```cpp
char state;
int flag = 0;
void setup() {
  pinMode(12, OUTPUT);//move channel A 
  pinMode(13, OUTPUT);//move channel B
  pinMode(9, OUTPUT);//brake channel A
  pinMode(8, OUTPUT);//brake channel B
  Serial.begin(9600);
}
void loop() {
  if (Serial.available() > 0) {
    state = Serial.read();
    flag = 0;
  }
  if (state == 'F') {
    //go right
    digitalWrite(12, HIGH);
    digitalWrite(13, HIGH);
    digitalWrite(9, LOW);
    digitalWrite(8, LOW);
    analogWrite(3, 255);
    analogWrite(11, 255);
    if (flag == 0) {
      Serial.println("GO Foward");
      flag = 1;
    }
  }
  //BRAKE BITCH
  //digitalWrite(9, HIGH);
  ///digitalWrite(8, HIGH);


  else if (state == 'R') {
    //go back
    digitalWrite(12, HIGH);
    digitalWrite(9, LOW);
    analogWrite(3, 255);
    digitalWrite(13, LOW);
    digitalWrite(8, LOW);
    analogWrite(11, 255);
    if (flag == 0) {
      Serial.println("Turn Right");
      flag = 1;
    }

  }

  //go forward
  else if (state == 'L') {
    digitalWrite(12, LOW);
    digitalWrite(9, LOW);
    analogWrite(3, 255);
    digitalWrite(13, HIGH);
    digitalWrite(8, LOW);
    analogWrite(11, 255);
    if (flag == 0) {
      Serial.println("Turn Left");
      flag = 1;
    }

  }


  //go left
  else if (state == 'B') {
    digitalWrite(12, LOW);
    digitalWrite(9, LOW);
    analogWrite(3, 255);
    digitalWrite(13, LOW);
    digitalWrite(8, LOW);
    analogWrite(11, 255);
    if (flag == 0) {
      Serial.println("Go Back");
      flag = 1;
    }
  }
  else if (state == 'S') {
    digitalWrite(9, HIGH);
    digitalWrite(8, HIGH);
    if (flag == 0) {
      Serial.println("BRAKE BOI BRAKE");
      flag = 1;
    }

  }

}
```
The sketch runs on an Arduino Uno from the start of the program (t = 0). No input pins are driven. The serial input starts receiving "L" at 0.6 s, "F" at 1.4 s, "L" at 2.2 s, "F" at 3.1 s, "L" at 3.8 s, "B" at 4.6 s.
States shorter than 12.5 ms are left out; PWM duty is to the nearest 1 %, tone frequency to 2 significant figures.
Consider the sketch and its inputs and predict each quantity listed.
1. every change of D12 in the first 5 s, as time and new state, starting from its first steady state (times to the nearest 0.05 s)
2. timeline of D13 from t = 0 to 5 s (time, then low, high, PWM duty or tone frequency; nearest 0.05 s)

0 s low; 1.4 s high; 2.2 s low; 3.1 s high; 3.8 s low
0 s low; 0.6 s high; 4.6 s low
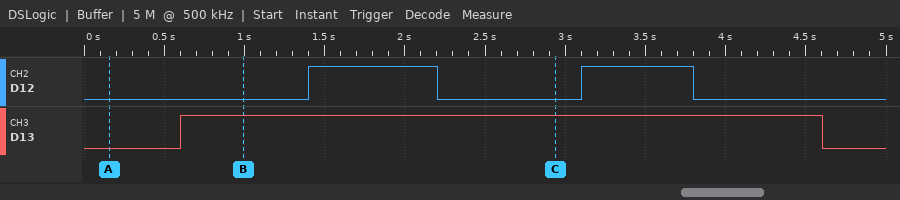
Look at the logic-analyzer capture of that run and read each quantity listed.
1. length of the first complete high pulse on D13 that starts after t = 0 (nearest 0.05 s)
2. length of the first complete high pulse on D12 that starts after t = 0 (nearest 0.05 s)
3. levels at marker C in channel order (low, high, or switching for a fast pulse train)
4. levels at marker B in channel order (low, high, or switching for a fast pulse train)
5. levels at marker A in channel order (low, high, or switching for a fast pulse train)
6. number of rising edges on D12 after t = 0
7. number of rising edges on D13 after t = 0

4.00 s
0.80 s
D12 low, D13 high
D12 low, D13 high
D12 low, D13 low
2
1
